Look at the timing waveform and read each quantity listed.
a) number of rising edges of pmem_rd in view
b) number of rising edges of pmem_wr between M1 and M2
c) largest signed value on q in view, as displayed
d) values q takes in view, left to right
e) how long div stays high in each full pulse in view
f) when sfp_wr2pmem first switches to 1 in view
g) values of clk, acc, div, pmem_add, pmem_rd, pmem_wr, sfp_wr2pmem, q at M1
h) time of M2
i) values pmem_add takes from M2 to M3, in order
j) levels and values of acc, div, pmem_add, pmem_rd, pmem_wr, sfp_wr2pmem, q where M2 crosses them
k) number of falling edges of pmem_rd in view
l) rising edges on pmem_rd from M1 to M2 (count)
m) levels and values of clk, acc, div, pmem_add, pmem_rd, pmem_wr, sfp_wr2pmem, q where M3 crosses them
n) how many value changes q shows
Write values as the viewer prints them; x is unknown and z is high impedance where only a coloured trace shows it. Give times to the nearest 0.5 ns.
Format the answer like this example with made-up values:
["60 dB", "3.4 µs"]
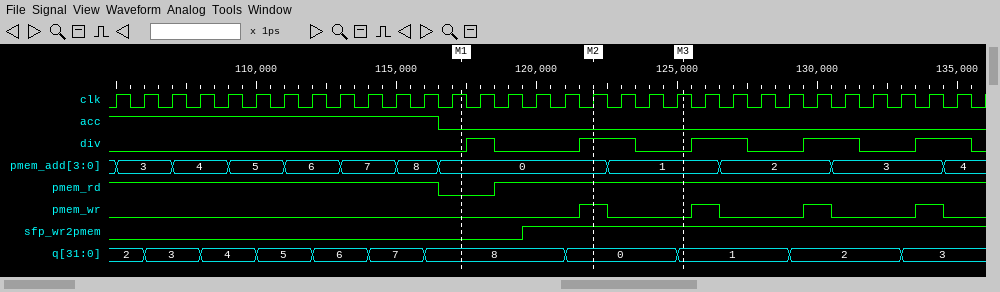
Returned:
["1", "1", "8", "2, 3, 4, 5, 6, 7, 8, 0, 1, 2, 3", "1 ns, 2 ns, 2 ns, 2 ns, 2 ns", "119.5 ns", "clk=1, acc=0, div=0, pmem_add=0, pmem_rd=0, pmem_wr=0, sfp_wr2pmem=0, q=8", "122 ns", "0, 1", "acc=0, div=1, pmem_add=0, pmem_rd=1, pmem_wr=1, sfp_wr2pmem=1, q=0", "1", "1", "clk=1, acc=0, div=0, pmem_add=1, pmem_rd=1, pmem_wr=0, sfp_wr2pmem=1, q=1", "10"]
